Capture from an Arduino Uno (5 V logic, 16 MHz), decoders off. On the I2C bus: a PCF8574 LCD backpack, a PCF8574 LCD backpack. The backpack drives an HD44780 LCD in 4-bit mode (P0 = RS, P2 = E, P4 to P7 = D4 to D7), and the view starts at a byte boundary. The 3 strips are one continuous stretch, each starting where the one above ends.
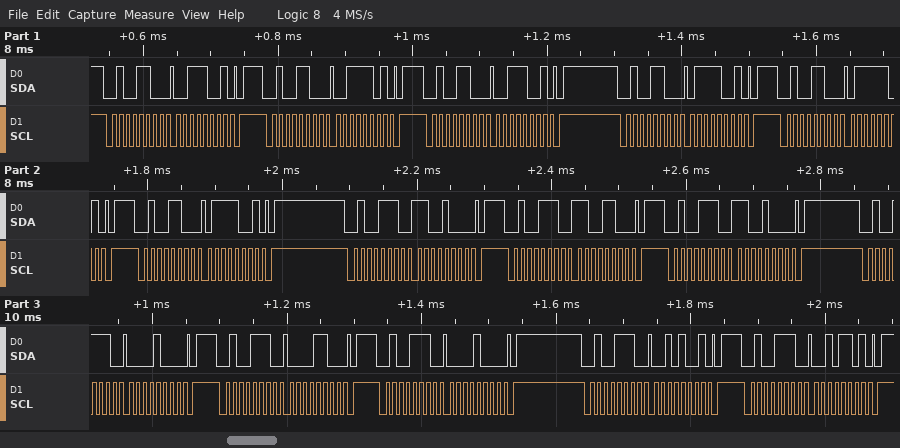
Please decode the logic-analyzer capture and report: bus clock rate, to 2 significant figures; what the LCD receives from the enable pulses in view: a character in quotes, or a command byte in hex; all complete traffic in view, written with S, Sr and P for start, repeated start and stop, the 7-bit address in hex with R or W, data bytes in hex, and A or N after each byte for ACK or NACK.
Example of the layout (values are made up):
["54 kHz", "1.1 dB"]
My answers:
["100 kHz", "'7' 0xC0", "S 26W A 39 A P S 26W A 3D A P S 26W A 39 A P S 26W A 79 A P S 26W A 7D A P S 26W A 79 A P S 27W A C8 A P S 27W A CC A P S 27W A C8 A P S 27W A 08 A P S 27W A 0C A P S 27W A 08 A P S 27W A 29 A P S 27W A 2D A P"]
